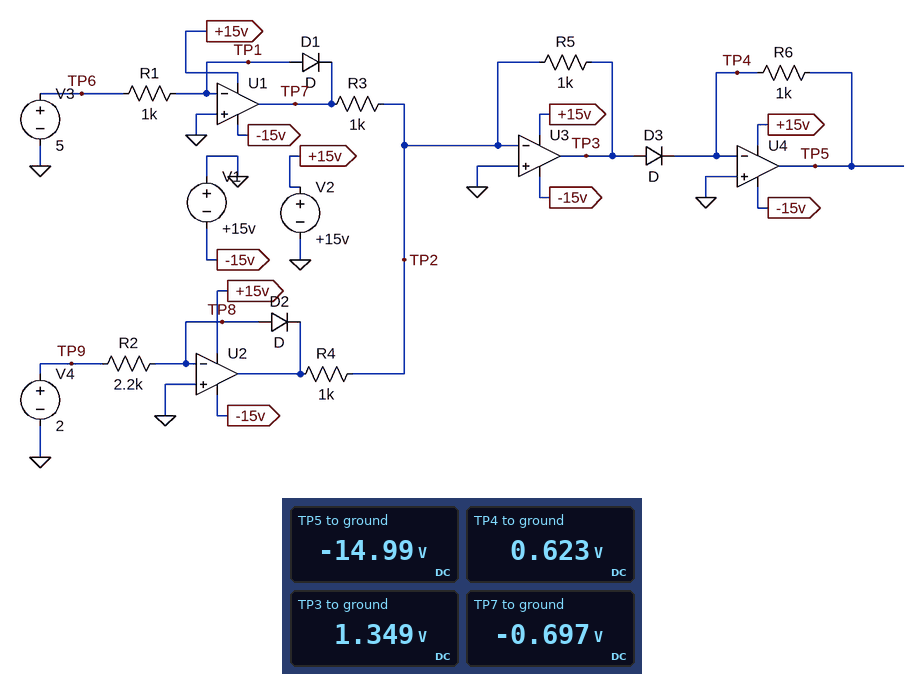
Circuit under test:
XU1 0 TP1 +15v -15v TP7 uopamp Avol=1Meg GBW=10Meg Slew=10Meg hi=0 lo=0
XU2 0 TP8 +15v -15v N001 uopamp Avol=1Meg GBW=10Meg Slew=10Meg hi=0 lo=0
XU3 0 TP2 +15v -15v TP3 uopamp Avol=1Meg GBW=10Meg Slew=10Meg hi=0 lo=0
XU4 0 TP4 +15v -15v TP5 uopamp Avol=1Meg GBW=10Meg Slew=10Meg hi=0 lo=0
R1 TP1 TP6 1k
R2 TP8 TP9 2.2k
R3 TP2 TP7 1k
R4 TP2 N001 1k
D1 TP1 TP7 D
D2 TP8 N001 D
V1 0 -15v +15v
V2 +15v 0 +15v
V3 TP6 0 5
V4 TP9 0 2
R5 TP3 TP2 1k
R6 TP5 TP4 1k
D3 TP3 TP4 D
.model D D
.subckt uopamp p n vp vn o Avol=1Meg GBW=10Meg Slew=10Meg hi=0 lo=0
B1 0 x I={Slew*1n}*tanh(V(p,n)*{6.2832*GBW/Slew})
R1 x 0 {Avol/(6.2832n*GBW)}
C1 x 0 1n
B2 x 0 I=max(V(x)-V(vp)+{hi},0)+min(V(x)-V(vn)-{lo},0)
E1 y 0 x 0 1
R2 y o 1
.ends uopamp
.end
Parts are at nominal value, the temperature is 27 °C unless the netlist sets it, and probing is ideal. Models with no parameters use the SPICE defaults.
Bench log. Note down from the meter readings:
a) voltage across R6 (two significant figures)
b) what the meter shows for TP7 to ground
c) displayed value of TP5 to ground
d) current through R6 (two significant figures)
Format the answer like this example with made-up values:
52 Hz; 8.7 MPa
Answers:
16 V; -0.697 V; -14.99 V; 16 mA
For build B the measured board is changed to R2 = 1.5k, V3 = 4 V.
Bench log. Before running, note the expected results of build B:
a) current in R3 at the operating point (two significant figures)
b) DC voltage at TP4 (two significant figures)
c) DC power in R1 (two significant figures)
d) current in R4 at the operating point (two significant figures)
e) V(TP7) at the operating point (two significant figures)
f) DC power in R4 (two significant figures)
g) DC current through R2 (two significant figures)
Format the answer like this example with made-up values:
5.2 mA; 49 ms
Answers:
690 µA; 630 mV; 16 mW; 660 µA; -690 mV; 440 µW; 1.3 mA
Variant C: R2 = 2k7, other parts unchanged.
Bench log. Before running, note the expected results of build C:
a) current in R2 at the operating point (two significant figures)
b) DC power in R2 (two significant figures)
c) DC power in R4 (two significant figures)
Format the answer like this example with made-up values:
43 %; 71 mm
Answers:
740 µA; 1.5 mW; 420 µW
